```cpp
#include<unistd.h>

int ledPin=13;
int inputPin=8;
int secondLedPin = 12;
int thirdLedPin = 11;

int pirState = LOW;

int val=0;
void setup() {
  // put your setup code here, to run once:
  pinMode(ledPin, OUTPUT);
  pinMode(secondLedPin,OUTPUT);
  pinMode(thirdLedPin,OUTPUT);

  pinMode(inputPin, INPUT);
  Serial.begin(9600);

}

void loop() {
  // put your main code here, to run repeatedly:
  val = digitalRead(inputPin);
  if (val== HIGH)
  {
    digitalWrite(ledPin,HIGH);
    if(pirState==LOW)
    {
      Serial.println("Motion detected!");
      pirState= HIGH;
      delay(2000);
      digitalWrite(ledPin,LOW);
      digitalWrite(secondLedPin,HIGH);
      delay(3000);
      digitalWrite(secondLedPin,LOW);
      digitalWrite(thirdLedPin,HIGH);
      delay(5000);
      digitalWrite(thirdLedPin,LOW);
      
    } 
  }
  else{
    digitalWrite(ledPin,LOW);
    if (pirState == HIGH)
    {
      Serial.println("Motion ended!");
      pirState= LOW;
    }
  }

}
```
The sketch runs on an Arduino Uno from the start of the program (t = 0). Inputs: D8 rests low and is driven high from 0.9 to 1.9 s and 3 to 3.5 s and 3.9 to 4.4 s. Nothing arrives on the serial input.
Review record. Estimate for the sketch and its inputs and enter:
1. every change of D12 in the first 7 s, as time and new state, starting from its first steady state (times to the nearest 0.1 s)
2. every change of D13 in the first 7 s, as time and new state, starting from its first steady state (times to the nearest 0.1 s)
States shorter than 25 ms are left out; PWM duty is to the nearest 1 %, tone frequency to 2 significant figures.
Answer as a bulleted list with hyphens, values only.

- 0 s low; 2.9 s high; 5.9 s low
- 0 s low; 0.9 s high; 2.9 s low
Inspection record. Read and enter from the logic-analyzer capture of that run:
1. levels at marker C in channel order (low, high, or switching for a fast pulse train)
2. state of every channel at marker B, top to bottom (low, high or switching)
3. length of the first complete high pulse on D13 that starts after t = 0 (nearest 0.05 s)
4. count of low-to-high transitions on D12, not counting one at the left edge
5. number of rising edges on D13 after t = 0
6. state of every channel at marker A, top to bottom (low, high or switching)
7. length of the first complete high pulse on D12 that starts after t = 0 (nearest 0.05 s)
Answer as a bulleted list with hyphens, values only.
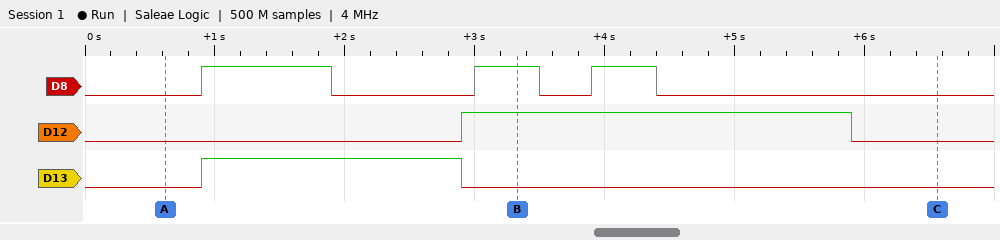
- D8 low, D12 low, D13 low
- D8 high, D12 high, D13 low
- 2.00 s
- 1
- 1
- D8 low, D12 low, D13 low
- 3.00 s
